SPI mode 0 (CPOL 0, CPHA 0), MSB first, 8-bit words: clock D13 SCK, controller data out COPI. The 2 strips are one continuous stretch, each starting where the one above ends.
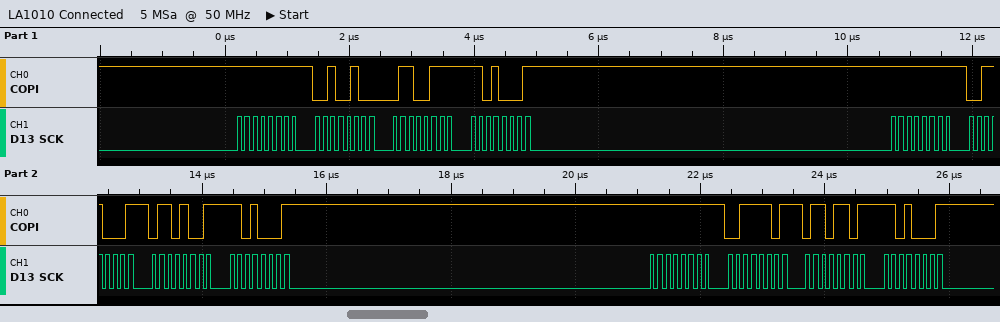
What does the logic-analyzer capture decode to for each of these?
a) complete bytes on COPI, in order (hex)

FF 24 67 D1 FF 31 69 D1 FF 3D 6D D1
